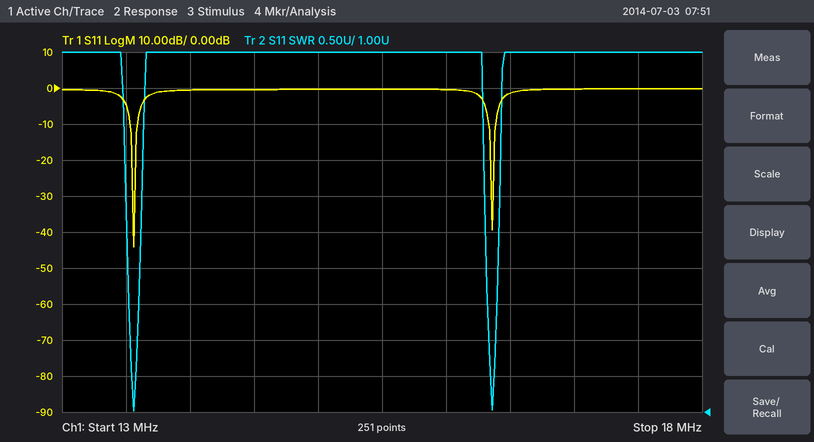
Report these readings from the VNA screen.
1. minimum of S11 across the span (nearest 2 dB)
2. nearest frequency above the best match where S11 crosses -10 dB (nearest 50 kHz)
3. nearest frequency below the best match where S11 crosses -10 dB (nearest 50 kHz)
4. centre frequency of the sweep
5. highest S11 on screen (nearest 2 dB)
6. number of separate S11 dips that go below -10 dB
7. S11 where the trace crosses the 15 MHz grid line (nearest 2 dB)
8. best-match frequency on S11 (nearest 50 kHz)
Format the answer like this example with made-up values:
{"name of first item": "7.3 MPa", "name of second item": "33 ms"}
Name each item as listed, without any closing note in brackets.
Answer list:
{"minimum of S11 across the span": "-44 dB", "nearest frequency above the best match where S11 crosses -10 dB": "13.60 MHz", "nearest frequency below the best match where S11 crosses -10 dB": "13.55 MHz", "centre frequency of the sweep": "15.5 MHz", "highest S11 on screen": "0 dB", "number of separate S11 dips that go below -10 dB": "2", "S11 where the trace crosses the 15 MHz grid line": "0 dB", "best-match frequency on S11": "13.55 MHz"}
